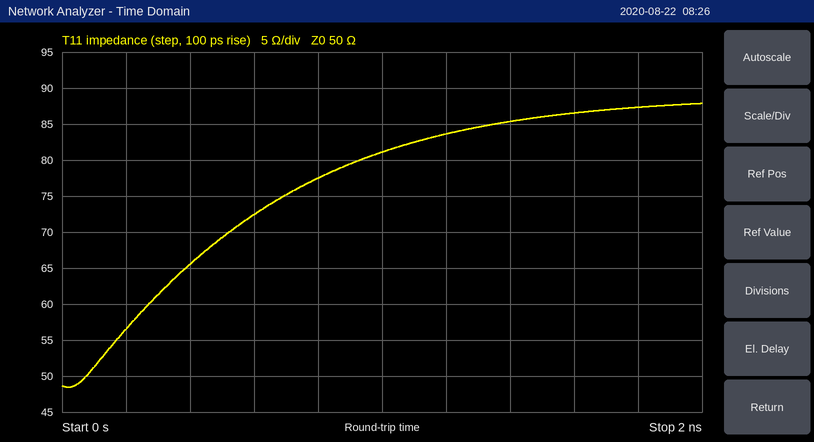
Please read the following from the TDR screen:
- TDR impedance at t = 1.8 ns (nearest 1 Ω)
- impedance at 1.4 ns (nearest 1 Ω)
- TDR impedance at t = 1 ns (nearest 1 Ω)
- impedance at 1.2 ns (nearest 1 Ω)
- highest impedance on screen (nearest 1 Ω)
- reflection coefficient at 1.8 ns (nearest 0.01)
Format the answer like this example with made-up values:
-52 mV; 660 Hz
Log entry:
87 Ω; 85 Ω; 81 Ω; 84 Ω; 88 Ω; +0.27
